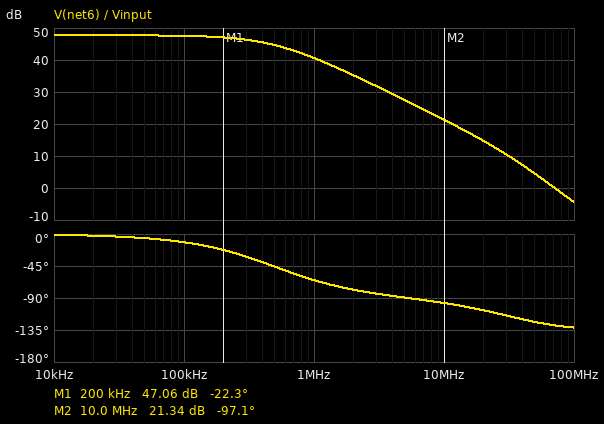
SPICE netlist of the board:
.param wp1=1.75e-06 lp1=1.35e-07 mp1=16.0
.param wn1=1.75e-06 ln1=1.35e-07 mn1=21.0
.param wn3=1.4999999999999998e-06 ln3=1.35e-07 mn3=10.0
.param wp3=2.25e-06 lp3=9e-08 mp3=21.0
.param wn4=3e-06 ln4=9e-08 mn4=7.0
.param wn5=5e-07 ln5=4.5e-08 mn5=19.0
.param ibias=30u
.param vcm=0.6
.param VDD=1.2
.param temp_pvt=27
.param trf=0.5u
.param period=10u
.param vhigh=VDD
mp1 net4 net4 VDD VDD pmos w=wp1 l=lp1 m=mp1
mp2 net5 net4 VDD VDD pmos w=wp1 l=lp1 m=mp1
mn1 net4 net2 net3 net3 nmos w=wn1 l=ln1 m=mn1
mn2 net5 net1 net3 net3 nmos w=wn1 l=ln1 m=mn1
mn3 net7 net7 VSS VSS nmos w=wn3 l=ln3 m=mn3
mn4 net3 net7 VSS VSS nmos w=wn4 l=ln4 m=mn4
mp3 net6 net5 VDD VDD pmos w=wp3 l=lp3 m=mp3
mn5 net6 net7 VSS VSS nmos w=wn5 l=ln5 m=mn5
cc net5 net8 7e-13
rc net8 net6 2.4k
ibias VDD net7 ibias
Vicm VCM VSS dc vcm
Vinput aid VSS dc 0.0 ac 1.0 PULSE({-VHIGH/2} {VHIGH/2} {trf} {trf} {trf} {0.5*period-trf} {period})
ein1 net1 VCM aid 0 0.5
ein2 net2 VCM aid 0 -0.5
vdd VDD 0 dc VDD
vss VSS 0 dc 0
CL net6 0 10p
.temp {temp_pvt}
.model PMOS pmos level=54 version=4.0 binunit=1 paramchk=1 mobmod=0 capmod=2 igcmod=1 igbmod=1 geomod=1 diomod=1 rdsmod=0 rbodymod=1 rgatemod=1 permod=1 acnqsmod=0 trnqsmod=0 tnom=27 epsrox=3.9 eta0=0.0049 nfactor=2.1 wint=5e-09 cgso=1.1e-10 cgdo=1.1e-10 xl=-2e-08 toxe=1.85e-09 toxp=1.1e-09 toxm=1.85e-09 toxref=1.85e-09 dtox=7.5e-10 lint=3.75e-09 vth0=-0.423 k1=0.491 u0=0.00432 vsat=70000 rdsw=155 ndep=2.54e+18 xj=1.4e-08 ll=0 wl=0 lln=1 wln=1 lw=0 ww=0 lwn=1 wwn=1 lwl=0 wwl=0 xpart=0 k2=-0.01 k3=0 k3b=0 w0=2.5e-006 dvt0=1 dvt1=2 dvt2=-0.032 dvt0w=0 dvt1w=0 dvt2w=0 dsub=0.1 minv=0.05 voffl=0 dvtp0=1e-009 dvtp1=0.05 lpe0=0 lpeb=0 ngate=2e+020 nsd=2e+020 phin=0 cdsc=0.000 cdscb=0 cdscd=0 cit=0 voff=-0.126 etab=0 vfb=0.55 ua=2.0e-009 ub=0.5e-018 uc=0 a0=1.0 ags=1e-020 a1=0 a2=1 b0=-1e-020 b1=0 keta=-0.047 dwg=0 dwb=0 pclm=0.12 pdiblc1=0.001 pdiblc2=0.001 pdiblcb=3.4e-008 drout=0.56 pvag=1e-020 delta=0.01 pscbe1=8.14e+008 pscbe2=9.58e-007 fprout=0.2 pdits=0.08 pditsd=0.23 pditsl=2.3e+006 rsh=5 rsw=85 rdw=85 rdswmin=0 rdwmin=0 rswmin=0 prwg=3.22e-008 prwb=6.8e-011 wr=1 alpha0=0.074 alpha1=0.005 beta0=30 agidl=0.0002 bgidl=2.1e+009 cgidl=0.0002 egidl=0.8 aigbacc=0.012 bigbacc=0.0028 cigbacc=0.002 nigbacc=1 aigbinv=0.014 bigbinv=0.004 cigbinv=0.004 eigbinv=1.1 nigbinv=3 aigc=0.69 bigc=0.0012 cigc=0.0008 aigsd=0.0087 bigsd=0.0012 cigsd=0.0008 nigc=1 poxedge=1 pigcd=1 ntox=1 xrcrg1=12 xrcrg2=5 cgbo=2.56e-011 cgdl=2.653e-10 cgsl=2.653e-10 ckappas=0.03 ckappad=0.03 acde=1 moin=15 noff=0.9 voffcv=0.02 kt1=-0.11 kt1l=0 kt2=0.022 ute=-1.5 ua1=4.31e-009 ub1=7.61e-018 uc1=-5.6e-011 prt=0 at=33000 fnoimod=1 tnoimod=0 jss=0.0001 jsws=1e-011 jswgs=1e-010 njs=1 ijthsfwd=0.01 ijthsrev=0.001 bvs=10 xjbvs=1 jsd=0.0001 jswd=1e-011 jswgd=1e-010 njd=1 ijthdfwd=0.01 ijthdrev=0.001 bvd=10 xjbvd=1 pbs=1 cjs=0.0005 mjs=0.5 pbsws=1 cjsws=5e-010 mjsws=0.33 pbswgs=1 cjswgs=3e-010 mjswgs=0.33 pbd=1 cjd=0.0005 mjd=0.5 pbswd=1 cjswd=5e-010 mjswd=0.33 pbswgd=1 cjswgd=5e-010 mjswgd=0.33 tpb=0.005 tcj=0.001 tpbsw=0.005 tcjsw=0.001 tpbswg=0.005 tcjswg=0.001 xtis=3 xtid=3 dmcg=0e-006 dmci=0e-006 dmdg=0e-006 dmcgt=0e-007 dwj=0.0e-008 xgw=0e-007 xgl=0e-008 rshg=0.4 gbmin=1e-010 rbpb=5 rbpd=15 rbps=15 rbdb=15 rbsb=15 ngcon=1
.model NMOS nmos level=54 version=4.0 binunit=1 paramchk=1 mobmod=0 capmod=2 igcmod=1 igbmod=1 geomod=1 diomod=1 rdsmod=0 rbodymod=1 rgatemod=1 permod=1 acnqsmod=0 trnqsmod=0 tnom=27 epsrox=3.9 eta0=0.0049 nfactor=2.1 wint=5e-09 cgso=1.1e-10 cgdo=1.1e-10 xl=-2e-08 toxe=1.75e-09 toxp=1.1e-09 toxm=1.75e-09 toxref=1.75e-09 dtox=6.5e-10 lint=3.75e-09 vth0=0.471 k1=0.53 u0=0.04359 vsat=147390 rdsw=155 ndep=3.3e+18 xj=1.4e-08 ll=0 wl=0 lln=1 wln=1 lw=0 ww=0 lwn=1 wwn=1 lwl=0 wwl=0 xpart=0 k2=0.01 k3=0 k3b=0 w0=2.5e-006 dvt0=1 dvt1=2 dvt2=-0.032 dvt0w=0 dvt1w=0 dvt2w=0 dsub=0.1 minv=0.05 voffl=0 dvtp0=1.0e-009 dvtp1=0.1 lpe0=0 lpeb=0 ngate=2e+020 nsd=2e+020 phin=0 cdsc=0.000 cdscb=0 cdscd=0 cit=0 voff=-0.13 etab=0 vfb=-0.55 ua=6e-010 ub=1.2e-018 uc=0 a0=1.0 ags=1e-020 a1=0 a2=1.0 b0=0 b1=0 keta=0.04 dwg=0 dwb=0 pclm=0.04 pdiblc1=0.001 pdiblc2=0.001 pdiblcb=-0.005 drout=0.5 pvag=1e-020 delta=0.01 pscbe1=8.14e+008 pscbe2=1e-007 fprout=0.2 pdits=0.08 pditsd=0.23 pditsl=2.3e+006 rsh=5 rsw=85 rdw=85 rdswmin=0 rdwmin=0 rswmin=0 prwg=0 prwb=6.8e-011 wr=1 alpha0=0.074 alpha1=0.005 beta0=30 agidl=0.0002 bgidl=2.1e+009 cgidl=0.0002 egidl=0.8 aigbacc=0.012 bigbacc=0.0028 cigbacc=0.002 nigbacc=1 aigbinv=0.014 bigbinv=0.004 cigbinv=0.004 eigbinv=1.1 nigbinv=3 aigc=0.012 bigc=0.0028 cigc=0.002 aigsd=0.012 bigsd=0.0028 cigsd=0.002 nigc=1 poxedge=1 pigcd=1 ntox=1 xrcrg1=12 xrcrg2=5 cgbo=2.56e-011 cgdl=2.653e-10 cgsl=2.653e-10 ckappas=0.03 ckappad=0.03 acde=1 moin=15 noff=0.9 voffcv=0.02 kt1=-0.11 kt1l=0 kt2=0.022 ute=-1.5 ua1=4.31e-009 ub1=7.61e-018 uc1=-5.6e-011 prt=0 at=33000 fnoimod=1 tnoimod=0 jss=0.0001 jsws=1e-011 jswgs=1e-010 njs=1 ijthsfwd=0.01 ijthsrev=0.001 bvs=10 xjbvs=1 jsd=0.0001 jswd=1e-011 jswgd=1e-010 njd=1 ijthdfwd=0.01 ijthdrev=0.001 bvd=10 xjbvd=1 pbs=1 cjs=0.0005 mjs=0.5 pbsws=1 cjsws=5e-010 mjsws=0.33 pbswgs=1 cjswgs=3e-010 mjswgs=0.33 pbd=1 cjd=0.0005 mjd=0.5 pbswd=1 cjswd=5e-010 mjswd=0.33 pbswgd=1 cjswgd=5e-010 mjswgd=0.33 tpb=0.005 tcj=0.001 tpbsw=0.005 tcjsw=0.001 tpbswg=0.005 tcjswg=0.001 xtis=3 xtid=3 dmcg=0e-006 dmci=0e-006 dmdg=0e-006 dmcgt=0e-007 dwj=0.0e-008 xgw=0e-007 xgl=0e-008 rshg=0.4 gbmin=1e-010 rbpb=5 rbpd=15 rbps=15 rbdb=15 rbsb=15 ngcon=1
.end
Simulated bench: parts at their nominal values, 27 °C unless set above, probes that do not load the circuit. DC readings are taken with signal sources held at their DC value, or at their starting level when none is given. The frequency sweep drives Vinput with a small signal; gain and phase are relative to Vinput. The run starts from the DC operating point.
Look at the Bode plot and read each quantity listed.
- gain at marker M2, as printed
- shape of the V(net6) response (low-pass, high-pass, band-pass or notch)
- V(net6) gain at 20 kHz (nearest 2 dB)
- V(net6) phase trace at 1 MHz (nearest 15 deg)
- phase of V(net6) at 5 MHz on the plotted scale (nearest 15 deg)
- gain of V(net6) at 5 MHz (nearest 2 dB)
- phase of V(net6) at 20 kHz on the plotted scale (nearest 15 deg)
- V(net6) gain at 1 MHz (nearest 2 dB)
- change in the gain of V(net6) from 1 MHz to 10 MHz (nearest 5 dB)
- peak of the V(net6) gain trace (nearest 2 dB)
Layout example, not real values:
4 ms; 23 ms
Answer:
21.34 dB; low-pass; 48 dB; -60 deg; -90 deg; 28 dB; 0 deg; 40 dB; -20 dB; 48 dB
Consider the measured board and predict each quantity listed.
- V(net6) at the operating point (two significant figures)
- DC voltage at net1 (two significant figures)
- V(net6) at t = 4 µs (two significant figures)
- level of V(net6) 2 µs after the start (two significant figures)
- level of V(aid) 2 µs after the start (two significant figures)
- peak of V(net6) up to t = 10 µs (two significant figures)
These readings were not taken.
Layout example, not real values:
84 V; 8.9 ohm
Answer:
110 mV; 600 mV; 1.1 V; 1.1 V; 600 mV; 1.1 V
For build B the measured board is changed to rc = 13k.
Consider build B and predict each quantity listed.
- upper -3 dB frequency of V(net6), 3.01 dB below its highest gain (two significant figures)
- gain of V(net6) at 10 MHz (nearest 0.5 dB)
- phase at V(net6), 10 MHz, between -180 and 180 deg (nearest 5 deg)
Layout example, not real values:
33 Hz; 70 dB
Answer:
480 kHz; 22.5 dB; -75 deg
